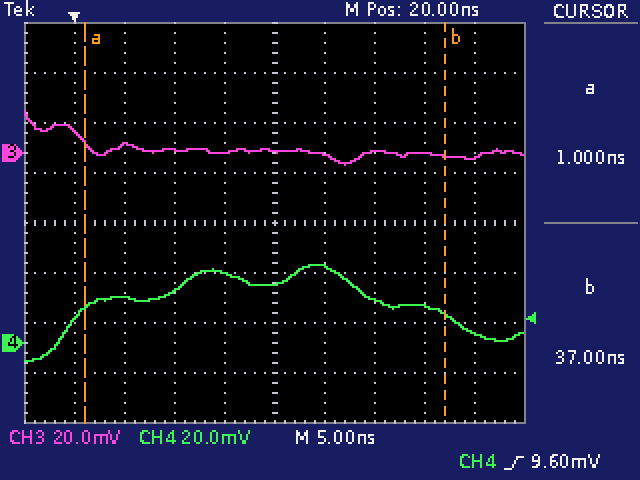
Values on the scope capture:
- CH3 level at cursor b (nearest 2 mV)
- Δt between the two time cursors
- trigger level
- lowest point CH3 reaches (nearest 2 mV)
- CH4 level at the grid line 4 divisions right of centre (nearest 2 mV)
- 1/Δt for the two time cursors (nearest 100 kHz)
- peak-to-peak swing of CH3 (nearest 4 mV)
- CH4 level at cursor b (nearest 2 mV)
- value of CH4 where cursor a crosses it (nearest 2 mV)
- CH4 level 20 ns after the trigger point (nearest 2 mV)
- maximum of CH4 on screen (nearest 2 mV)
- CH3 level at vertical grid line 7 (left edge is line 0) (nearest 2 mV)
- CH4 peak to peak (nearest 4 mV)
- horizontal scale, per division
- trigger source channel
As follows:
-2 mV
36.0 ns
9.60 mV
-4 mV
4 mV
27.8 MHz
20 mV
12 mV
14 mV
24 mV
32 mV
0 mV
40 mV
5 ns
CH4
